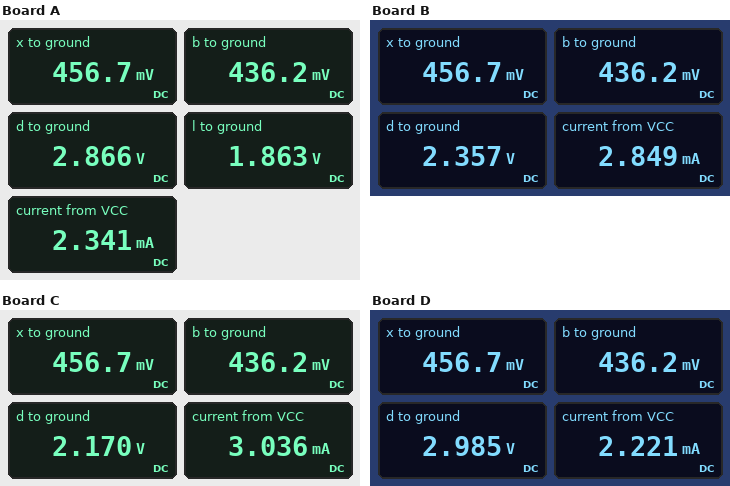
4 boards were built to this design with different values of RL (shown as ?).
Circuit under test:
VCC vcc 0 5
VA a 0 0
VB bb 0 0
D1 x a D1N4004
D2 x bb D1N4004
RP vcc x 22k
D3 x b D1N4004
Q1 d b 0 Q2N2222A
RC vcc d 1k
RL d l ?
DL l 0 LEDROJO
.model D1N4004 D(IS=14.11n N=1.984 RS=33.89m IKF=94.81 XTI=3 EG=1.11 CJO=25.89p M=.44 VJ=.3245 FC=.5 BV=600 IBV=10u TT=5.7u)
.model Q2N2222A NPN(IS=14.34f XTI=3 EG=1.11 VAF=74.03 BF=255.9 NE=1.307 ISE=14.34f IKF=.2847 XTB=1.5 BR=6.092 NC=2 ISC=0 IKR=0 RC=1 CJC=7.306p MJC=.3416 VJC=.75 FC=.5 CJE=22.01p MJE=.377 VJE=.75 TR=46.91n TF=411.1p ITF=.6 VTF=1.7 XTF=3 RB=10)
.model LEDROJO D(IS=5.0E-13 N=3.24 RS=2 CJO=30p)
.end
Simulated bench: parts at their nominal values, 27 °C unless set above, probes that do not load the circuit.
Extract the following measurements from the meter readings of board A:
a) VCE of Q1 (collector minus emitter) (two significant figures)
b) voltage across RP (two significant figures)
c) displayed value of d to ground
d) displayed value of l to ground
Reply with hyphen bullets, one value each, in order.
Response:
- 2.9 V
- 4.5 V
- 2.866 V
- 1.863 V
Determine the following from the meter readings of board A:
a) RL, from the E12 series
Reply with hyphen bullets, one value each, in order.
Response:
- 470 Ω
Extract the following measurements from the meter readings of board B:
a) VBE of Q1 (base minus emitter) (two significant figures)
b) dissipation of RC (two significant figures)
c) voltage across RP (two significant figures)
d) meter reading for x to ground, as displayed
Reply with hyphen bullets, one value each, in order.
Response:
- 440 mV
- 7.0 mW
- 4.5 V
- 456.7 mV
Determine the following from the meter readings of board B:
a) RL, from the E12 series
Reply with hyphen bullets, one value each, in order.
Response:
- 180 Ω
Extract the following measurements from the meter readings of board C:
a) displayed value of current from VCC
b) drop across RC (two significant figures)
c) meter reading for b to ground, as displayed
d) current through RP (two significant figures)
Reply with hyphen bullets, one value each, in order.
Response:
- 3.036 mA
- 2.8 V
- 436.2 mV
- 210 µA
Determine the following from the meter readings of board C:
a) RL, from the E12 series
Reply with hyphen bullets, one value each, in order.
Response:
- 100 Ω
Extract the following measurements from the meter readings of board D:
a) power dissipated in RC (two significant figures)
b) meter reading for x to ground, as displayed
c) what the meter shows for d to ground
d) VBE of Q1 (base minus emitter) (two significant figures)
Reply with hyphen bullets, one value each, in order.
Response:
- 4.1 mW
- 456.7 mV
- 2.985 V
- 440 mV
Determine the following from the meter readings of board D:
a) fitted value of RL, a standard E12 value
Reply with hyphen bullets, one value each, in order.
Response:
- 560 Ω
